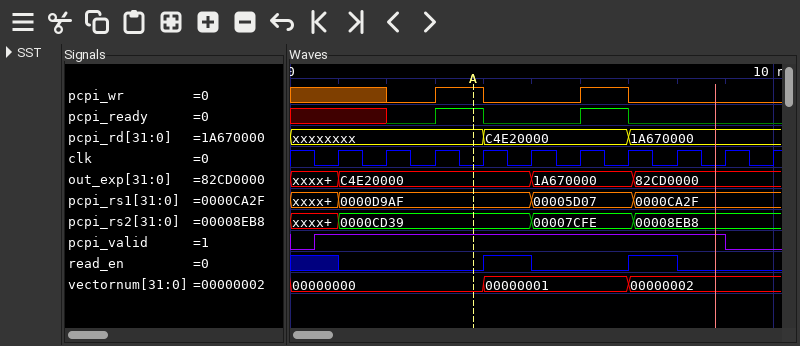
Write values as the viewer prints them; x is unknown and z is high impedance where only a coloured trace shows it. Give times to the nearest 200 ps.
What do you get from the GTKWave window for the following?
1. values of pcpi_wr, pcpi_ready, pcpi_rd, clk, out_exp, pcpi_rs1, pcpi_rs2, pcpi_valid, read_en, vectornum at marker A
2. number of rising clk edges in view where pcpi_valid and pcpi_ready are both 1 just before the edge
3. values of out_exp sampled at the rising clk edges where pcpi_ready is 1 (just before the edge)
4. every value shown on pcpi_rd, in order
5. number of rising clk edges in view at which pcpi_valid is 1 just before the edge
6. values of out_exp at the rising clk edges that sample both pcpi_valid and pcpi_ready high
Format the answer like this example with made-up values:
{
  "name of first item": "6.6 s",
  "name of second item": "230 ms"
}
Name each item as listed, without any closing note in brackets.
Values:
{
  "values of pcpi_wr, pcpi_ready, pcpi_rd, clk, out_exp, pcpi_rs1, pcpi_rs2, pcpi_valid, read_en, vectornum at marker A": "pcpi_wr=1, pcpi_ready=1, pcpi_rd=xxxxxxxx, clk=0, out_exp=C4E20000, pcpi_rs1=0000D9AF, pcpi_rs2=0000CD39, pcpi_valid=1, read_en=0, vectornum=00000000",
  "number of rising clk edges in view where pcpi_valid and pcpi_ready are both 1 just before the edge": "2",
  "values of out_exp sampled at the rising clk edges where pcpi_ready is 1": "C4E20000, 1A670000",
  "every value shown on pcpi_rd, in order": "xxxxxxxx, C4E20000, 1A670000",
  "number of rising clk edges in view at which pcpi_valid is 1 just before the edge": "9",
  "values of out_exp at the rising clk edges that sample both pcpi_valid and pcpi_ready high": "C4E20000, 1A670000"
}
